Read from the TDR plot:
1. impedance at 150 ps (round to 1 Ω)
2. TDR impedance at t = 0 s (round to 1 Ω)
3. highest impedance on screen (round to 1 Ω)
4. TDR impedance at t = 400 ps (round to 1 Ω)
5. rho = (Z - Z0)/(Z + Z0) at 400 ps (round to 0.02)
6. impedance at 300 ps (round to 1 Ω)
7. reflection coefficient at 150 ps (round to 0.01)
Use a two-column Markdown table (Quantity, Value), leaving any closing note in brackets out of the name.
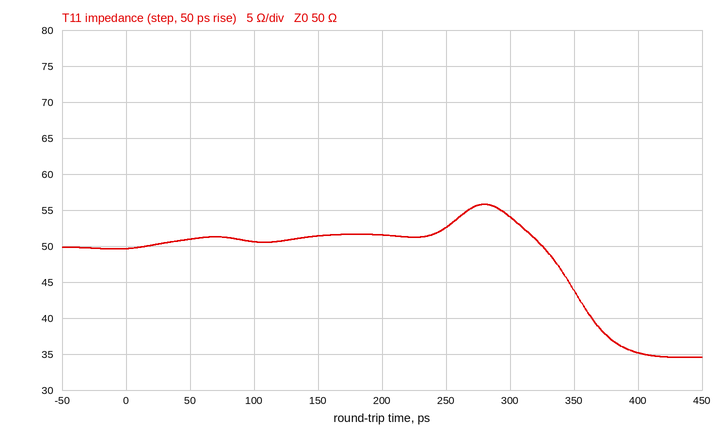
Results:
| Quantity | Value |
|---|---|
| impedance at 150 ps | 51 Ω |
| TDR impedance at t = 0 s | 50 Ω |
| highest impedance on screen | 56 Ω |
| TDR impedance at t = 400 ps | 35 Ω |
| rho = (Z - Z0)/(Z + Z0) at 400 ps | -0.18 |
| impedance at 300 ps | 54 Ω |
| reflection coefficient at 150 ps | +0.01 |
